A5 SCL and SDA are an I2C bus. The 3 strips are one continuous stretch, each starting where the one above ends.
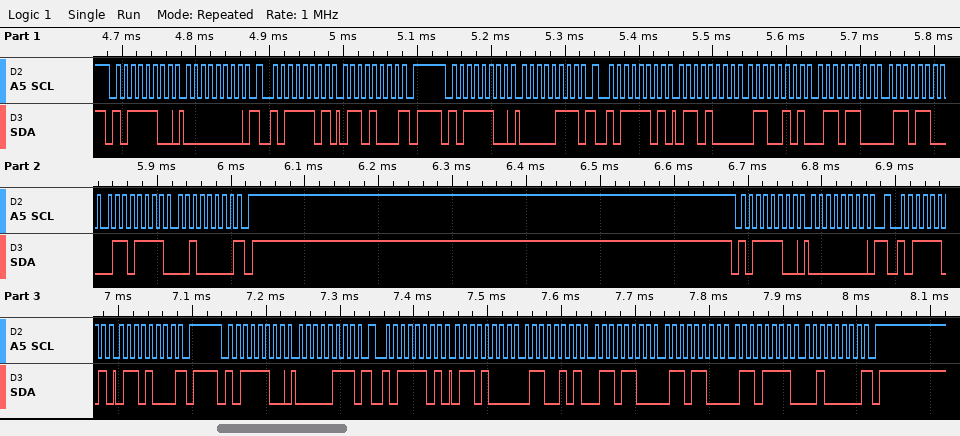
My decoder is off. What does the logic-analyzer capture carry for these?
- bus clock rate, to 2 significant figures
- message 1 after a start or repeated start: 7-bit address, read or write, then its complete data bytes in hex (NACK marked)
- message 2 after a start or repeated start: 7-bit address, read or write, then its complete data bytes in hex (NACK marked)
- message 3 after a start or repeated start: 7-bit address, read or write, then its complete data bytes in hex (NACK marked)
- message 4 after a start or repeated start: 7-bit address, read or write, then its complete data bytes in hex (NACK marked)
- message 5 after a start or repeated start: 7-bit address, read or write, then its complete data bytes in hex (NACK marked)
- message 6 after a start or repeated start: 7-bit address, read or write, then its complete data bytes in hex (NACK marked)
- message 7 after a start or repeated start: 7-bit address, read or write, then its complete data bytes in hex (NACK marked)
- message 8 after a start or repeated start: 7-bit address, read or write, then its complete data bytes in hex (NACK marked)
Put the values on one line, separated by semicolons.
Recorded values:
100 kHz; 0x5E write: 00; 0x5E read: 68 NACK; 0x5E write: 07; 0x5E read: 68 65 6C 6C 6F 20 NACK; 0x5E write: 00; 0x5E read: 68 NACK; 0x5E write: 07; 0x5E read: 68 65 6C 6C 6F 20 NACK
